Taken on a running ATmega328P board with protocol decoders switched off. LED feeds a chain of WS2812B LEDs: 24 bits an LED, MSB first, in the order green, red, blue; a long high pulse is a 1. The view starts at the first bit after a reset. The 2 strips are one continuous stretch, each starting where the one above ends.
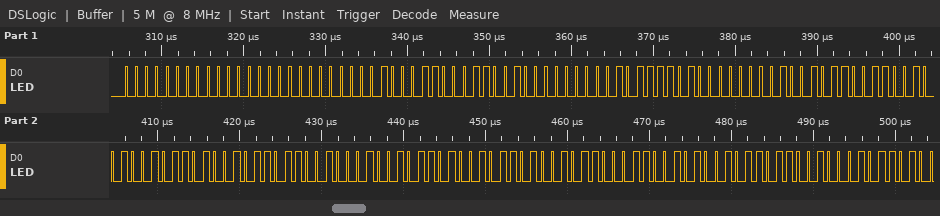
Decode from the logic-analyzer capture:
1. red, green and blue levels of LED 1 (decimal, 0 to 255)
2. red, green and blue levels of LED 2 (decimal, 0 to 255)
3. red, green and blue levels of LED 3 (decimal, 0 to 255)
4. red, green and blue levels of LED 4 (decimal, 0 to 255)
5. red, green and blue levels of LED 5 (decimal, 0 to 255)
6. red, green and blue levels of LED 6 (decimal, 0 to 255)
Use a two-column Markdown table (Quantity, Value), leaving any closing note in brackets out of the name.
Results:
| Quantity | Value |
|---|---|
| red, green and blue levels of LED 1 | 0, 0, 0 |
| red, green and blue levels of LED 2 | 50, 70, 0 |
| red, green and blue levels of LED 3 | 0, 189, 150 |
| red, green and blue levels of LED 4 | 150, 100, 150 |
| red, green and blue levels of LED 5 | 150, 200, 150 |
| red, green and blue levels of LED 6 | 50, 150, 150 |
